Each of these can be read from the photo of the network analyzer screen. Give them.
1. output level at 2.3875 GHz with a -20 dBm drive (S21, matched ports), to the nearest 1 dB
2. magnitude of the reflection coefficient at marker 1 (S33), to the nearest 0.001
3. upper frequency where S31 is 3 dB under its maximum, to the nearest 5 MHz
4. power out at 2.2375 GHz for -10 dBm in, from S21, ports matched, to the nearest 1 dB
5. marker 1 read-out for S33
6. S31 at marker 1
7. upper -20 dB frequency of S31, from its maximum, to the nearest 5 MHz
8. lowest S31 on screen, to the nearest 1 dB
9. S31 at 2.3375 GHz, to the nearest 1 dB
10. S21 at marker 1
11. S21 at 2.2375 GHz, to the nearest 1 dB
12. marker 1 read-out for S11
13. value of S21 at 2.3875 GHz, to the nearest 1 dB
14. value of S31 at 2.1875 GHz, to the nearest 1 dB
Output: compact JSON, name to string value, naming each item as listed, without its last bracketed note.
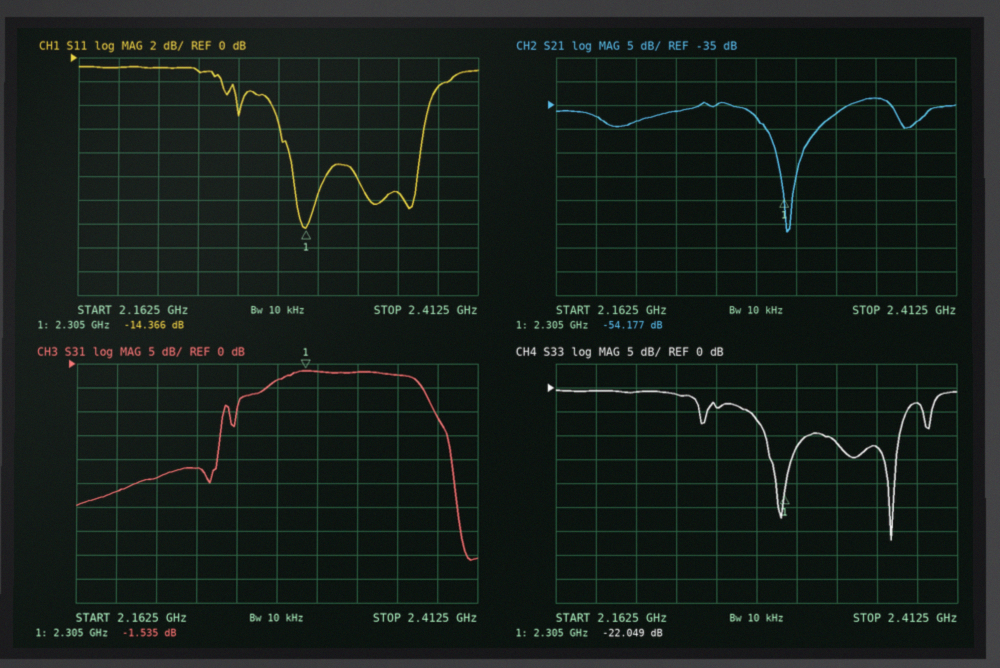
{"output level at 2.3875 GHz with a -20 dBm drive (S21, matched ports), to the nearest 1 dB": "-59 dBm", "magnitude of the reflection coefficient at marker 1 (S33), to the nearest 0.001": "0.079", "upper frequency where S31 is 3 dB under its maximum, to the nearest 5 MHz": "2.375 GHz", "power out at 2.2375 GHz for -10 dBm in, from S21, ports matched, to the nearest 1 dB": "-46 dBm", "marker 1 read-out for S33": "-22.049 dB", "S31 at marker 1": "-1.535 dB", "upper -20 dB frequency of S31, from its maximum, to the nearest 5 MHz": "2.395 GHz", "lowest S31 on screen, to the nearest 1 dB": "-41 dB", "S31 at 2.3375 GHz, to the nearest 1 dB": "-2 dB", "S21 at marker 1": "-54.177 dB", "S21 at 2.2375 GHz, to the nearest 1 dB": "-36 dB", "marker 1 read-out for S11": "-14.366 dB", "value of S21 at 2.3875 GHz, to the nearest 1 dB": "-39 dB", "value of S31 at 2.1875 GHz, to the nearest 1 dB": "-27 dB"}
